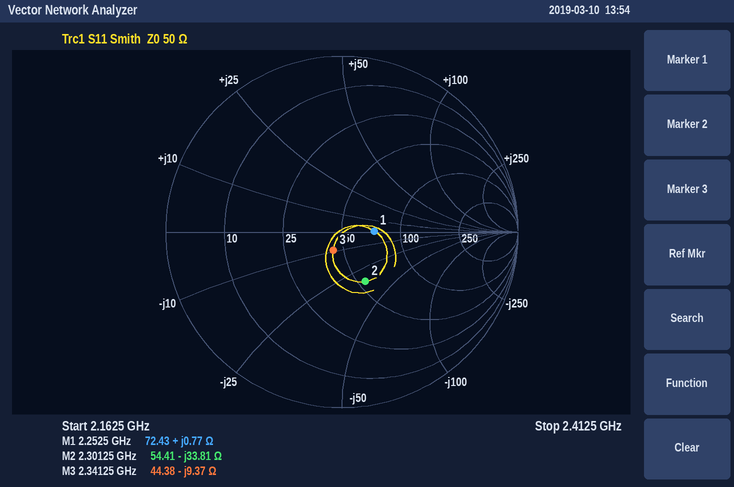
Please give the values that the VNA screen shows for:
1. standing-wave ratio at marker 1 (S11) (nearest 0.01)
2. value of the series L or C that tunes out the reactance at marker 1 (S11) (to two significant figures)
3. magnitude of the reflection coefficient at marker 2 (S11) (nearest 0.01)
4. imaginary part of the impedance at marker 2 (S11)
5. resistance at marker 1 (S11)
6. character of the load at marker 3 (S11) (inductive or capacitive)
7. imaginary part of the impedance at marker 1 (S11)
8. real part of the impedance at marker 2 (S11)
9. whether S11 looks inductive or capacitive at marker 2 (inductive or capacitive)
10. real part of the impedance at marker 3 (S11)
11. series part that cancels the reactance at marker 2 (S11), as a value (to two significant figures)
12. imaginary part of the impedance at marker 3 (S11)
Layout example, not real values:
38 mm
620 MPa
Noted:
1.45
92 pF
0.31
-33.81 Ω
72.43 Ω
capacitive
+0.77 Ω
54.41 Ω
capacitive
44.38 Ω
2.3 nH
-9.37 Ω
